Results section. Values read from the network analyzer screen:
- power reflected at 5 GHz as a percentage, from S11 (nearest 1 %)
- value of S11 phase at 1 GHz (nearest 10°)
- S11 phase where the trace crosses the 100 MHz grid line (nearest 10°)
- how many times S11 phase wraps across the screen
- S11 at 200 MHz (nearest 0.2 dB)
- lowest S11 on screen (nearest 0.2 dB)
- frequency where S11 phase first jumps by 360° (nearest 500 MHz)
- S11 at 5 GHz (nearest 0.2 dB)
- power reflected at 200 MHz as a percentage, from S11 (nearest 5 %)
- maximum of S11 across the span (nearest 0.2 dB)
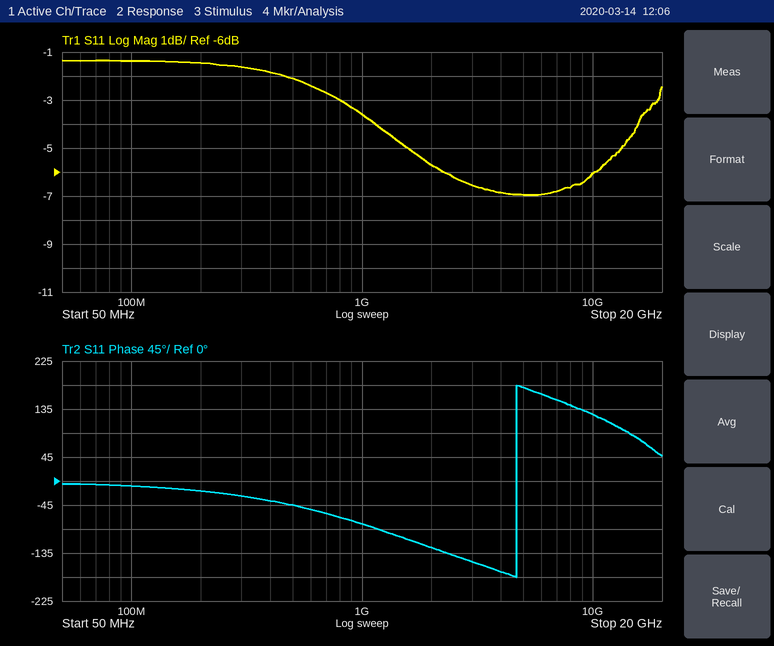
20 %
-80°
-10°
1
-1.4 dB
-7.0 dB
4.5 GHz
-7.0 dB
70 %
-1.4 dB
